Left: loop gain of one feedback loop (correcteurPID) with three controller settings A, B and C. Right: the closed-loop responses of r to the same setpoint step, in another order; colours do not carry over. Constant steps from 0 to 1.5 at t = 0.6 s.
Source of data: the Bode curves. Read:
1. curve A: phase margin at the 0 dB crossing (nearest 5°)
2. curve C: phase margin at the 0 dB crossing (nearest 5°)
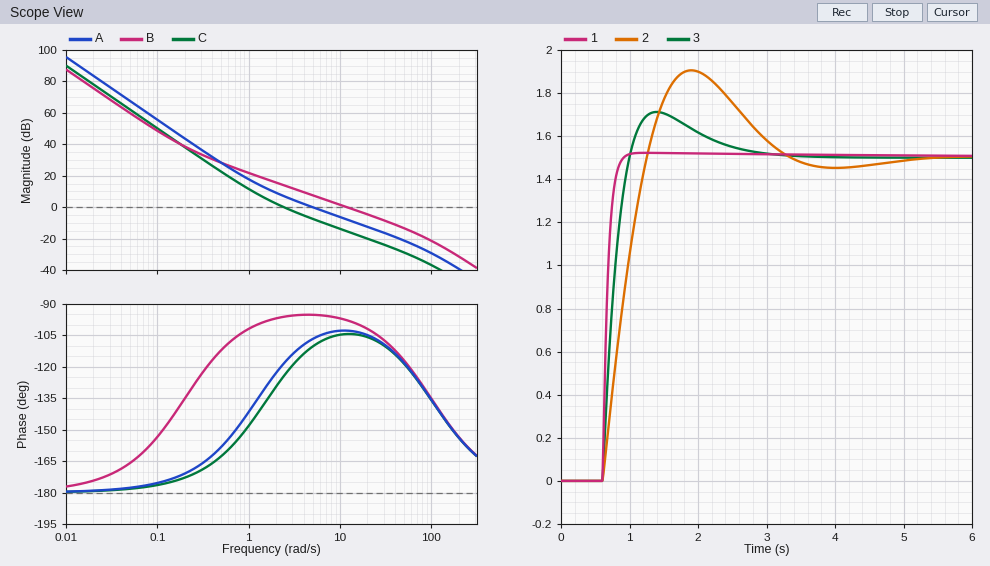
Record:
75°
55°
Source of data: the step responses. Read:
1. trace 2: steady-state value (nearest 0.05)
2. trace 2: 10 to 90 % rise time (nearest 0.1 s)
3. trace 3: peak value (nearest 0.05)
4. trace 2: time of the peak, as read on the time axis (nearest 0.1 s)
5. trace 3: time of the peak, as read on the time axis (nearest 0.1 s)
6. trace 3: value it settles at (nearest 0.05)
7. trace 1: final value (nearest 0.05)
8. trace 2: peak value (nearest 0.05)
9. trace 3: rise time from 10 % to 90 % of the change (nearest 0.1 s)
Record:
1.50
0.5 s
1.70
1.9 s
1.4 s
1.50
1.50
1.90
0.3 s
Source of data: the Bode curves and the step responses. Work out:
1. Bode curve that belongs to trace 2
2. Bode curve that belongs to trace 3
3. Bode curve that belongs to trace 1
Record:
C
A
B
